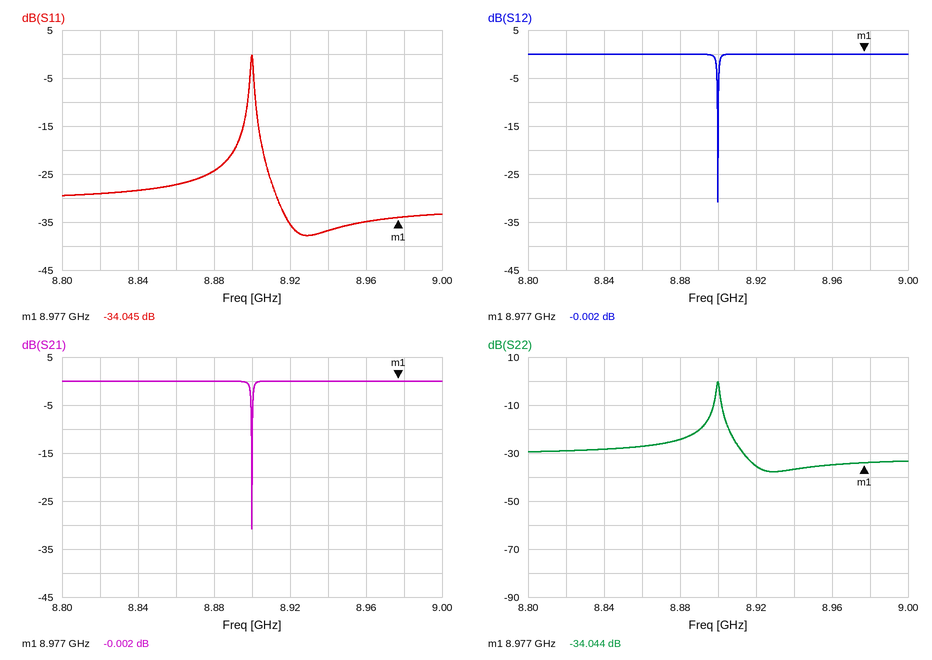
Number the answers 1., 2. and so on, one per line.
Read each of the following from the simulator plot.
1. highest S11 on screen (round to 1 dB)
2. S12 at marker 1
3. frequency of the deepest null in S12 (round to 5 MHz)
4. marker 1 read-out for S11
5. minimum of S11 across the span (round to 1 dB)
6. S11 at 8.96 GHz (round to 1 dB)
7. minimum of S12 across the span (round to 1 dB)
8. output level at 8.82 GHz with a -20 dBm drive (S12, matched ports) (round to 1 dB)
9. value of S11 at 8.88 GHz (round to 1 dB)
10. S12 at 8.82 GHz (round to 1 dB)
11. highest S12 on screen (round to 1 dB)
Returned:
1. 0 dB
2. -0.002 dB
3. 8.900 GHz
4. -34.045 dB
5. -38 dB
6. -35 dB
7. -31 dB
8. -20 dBm
9. -24 dB
10. 0 dB
11. 0 dB
